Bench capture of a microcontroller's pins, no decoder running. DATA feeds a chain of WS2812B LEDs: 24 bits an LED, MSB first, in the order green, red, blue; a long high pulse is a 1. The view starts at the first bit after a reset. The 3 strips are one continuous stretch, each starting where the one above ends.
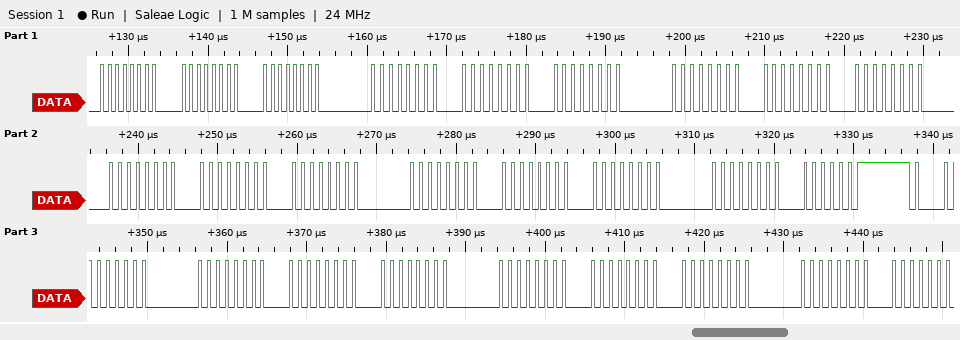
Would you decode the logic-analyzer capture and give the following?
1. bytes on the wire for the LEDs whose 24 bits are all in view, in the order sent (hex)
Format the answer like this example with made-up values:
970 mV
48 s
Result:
00 00 00 00 00 00 00 00 00 00 00 00 00 00 00 00 02 00 00 00 00 00 00 00
